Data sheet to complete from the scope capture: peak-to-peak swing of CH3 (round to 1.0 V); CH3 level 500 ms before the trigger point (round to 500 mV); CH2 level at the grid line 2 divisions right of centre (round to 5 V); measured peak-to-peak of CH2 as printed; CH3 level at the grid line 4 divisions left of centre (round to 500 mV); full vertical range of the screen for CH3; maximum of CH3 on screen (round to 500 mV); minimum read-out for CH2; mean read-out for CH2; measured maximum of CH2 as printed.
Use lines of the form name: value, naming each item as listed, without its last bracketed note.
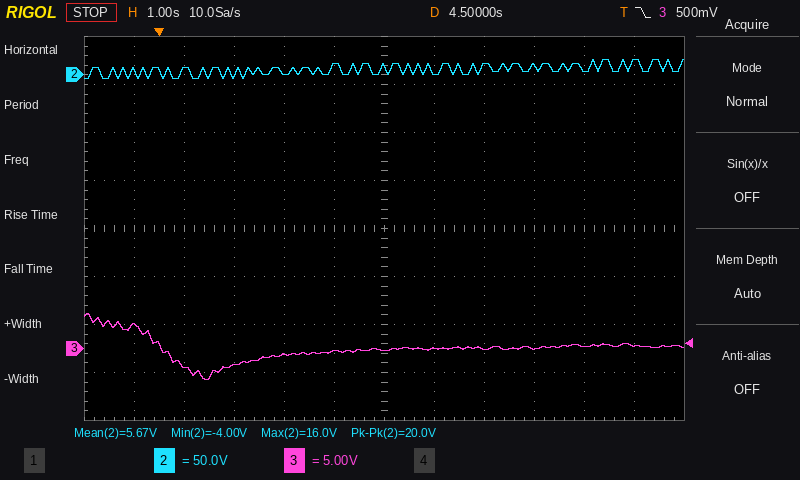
peak-to-peak swing of CH3: 7.0 V
CH3 level 500 ms before the trigger point: 2.5 V
CH2 level at the grid line 2 divisions right of centre: 10 V
measured peak-to-peak of CH2 as printed: 20.0 V
CH3 level at the grid line 4 divisions left of centre: -2.0 V
full vertical range of the screen for CH3: 40 V
maximum of CH3 on screen: 3.5 V
minimum read-out for CH2: -4.00 V
mean read-out for CH2: 5.67 V
measured maximum of CH2 as printed: 16.0 V
